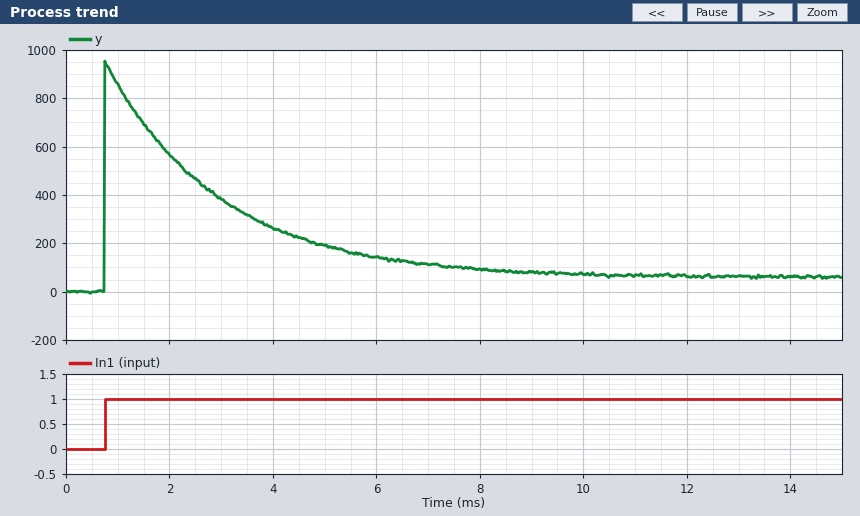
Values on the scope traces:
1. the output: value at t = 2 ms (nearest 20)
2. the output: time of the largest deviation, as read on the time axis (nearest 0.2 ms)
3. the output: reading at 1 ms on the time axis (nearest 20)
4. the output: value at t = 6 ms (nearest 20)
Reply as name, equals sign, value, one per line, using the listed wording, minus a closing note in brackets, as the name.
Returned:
the output: value at t = 2 ms = 560
the output: time of the largest deviation, as read on the time axis = 0.8 ms
the output: reading at 1 ms on the time axis = 860
the output: value at t = 6 ms = 140
